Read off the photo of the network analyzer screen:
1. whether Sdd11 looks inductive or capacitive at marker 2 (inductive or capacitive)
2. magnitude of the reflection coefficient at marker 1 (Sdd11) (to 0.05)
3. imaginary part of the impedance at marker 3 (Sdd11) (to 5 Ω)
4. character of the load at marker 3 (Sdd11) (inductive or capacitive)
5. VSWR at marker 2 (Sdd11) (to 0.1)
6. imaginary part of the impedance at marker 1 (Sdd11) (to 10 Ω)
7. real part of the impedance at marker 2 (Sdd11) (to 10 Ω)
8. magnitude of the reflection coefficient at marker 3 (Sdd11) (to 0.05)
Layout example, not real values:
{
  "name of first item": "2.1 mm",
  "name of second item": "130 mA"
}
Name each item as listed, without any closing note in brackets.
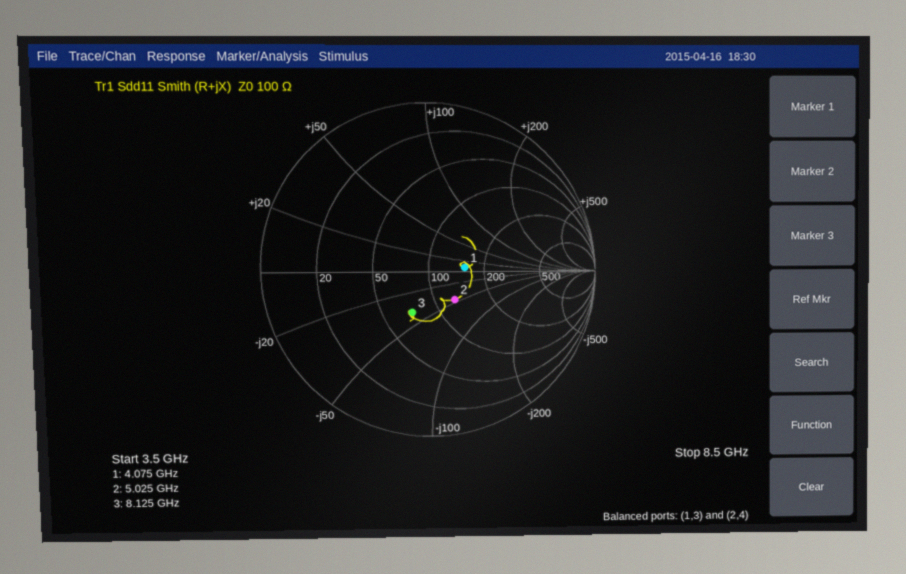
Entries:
{
  "whether Sdd11 looks inductive or capacitive at marker 2": "capacitive",
  "magnitude of the reflection coefficient at marker 1 (Sdd11)": "0.20",
  "imaginary part of the impedance at marker 3 (Sdd11)": "-40 Ω",
  "character of the load at marker 3 (Sdd11)": "capacitive",
  "VSWR at marker 2 (Sdd11)": "1.6",
  "imaginary part of the impedance at marker 1 (Sdd11)": "+10 Ω",
  "real part of the impedance at marker 2 (Sdd11)": "130 Ω",
  "magnitude of the reflection coefficient at marker 3 (Sdd11)": "0.25"
}
